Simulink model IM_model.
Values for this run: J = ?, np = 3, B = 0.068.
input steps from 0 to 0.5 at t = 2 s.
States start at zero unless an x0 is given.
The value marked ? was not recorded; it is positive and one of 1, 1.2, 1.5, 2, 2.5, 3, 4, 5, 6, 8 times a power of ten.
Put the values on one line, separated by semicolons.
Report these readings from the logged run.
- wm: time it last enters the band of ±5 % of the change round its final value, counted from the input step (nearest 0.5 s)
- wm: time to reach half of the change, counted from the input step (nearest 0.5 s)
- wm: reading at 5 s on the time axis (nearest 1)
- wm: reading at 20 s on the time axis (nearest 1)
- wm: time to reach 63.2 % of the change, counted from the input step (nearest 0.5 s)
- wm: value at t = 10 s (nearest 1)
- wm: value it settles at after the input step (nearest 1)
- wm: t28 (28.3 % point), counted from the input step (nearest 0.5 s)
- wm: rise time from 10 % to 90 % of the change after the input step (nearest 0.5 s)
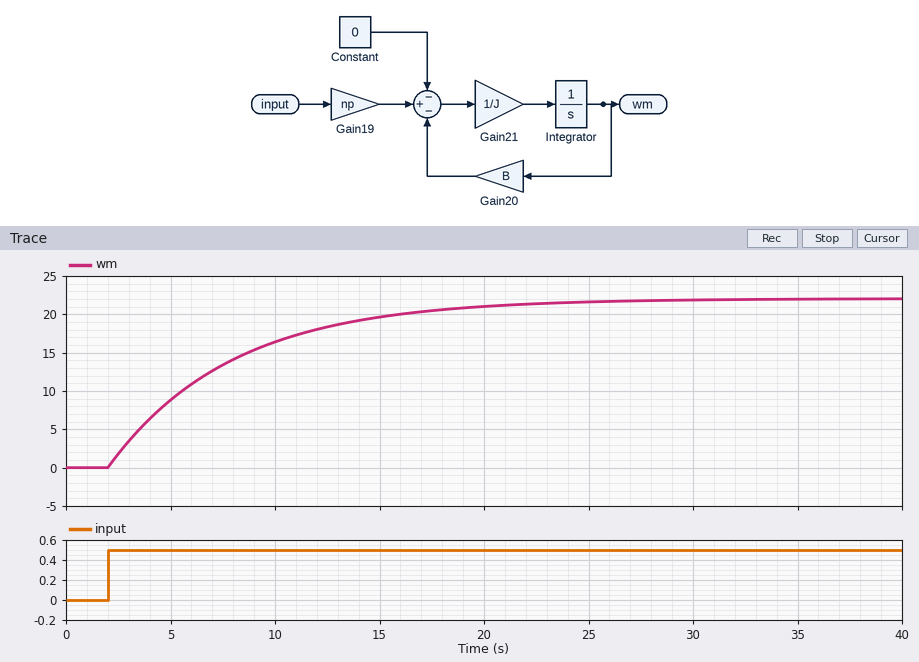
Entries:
17.5 s; 4.0 s; 9; 21; 6.0 s; 16; 22; 2.0 s; 13.0 s
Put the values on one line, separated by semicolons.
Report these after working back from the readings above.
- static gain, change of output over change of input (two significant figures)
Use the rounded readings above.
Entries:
44
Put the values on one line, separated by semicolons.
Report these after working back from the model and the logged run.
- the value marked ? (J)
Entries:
0.4
